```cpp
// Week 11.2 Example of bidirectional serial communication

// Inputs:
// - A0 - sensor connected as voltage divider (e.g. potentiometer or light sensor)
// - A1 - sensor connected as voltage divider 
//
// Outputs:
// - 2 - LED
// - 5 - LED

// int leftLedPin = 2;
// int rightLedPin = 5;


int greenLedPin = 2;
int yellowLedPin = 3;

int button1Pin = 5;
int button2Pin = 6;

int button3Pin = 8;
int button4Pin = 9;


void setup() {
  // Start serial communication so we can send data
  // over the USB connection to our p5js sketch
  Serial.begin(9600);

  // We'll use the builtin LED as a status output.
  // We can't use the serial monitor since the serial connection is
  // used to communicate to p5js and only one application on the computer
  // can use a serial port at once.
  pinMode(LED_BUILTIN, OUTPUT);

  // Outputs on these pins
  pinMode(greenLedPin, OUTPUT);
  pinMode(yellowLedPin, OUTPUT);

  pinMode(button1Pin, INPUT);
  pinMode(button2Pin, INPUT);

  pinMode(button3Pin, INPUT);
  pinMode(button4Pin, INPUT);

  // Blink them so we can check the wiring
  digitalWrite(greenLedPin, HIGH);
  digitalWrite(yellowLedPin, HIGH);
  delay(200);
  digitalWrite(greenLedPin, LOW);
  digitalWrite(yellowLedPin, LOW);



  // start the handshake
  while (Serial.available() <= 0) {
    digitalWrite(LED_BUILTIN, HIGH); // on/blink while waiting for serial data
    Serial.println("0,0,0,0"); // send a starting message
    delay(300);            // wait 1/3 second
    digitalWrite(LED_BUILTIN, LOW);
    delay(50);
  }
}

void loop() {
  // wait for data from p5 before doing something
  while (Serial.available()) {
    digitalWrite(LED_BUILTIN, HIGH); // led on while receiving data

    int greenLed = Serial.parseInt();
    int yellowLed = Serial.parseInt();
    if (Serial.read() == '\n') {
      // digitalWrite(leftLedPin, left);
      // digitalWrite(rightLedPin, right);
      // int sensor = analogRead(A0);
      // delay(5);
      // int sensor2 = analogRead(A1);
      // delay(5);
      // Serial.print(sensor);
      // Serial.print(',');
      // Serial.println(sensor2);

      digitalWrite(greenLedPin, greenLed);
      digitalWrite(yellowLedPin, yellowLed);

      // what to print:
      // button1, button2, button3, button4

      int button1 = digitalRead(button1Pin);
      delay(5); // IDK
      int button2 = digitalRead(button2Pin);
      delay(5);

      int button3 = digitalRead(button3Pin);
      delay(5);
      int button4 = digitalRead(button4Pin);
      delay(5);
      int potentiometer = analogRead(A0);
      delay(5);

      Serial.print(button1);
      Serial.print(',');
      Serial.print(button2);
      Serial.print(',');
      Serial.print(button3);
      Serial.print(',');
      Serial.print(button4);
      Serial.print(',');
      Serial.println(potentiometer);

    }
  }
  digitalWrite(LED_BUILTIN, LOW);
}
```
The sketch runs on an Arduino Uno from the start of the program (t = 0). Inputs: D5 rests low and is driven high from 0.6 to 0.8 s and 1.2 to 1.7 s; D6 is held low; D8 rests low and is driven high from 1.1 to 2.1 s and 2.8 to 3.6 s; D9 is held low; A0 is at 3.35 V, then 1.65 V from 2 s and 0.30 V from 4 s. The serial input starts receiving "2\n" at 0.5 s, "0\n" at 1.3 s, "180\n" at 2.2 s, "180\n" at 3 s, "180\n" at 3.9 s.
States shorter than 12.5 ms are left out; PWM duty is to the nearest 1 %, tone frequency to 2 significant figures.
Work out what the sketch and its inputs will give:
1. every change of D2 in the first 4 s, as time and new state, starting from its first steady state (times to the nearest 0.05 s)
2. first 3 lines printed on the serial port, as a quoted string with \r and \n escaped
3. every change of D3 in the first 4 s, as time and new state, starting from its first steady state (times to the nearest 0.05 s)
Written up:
0 s high; 0.2 s low; 1.3 s high
"0,0,0,0\r\n1,0,1,0,686\r\n0,0,1,0,337\r\n"
0 s high; 0.2 s low; 3 s high
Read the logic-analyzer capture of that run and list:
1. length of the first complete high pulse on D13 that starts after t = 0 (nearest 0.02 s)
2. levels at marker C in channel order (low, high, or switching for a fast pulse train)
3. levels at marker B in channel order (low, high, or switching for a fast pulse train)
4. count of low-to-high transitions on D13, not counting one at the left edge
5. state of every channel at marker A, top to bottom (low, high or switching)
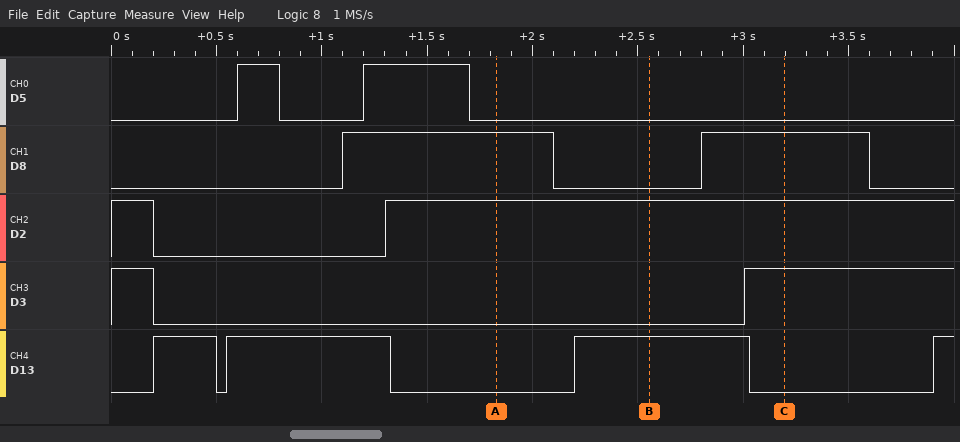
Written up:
0.30 s
D5 low, D8 high, D2 high, D3 high, D13 low
D5 low, D8 low, D2 high, D3 low, D13 high
4
D5 low, D8 high, D2 high, D3 low, D13 low
